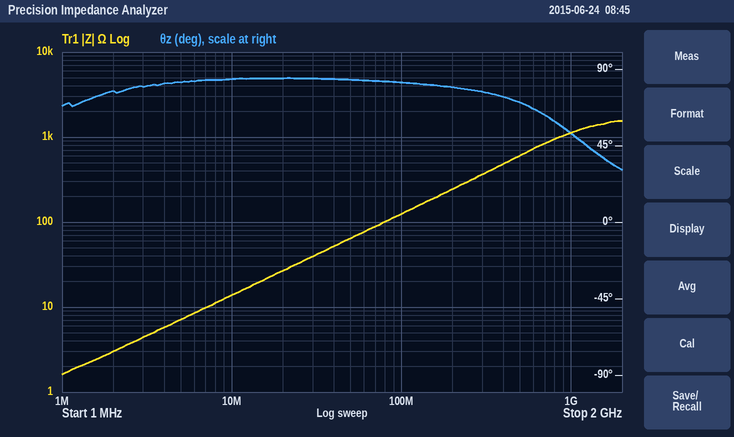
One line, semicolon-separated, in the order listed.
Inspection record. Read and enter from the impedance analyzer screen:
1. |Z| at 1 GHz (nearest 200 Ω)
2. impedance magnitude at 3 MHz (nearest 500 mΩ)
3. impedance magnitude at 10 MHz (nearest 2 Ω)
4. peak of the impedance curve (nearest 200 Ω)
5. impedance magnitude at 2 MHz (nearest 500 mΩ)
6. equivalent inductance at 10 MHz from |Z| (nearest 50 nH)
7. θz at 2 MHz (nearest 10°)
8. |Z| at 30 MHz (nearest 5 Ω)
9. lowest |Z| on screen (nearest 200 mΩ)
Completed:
1.2 kΩ; 4.5 Ω; 14 Ω; 1.6 kΩ; 3.0 Ω; 200 nH; 80°; 40 Ω; 1.6 Ω
